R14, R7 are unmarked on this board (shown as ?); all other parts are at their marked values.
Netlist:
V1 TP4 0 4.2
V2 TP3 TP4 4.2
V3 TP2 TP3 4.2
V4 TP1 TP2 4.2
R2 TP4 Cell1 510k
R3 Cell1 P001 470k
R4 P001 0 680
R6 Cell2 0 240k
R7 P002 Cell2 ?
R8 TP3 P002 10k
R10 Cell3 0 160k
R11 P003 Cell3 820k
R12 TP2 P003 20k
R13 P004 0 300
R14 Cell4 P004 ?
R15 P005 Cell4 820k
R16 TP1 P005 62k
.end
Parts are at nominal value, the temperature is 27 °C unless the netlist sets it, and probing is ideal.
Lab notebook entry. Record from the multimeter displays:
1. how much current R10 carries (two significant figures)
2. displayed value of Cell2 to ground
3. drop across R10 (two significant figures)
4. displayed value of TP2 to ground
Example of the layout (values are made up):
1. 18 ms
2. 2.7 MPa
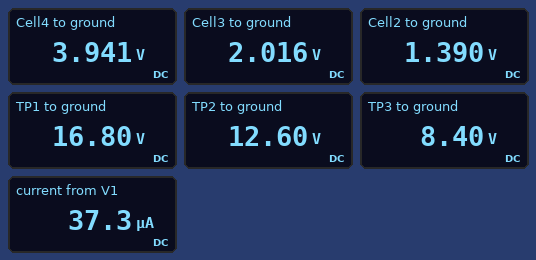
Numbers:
1. 13 µA
2. 1.390 V
3. 2.0 V
4. 12.60 V
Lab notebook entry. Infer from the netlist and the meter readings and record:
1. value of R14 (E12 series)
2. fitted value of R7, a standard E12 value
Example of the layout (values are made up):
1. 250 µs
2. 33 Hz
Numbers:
1. 270 kΩ
2. 1.2 MΩ
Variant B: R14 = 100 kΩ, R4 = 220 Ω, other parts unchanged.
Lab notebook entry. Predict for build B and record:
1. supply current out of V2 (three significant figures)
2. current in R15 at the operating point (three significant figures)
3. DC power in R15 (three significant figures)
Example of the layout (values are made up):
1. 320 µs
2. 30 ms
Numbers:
1. 35.5 µA
2. 17.1 µA
3. 240 µW
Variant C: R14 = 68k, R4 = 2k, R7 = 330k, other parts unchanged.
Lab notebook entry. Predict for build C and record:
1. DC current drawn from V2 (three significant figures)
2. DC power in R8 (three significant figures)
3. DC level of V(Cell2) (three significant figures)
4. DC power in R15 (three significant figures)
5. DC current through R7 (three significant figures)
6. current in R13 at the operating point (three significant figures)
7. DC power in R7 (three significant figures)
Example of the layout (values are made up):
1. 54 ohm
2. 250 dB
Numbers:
1. 44.8 µA
2. 2.10 µW
3. 3.48 V
4. 256 µW
5. 14.5 µA
6. 17.7 µA
7. 69.2 µW
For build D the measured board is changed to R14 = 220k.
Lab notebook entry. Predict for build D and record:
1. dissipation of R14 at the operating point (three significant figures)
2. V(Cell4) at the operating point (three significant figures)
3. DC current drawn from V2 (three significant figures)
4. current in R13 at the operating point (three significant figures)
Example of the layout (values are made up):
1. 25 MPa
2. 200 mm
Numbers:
1. 51.1 µW
2. 3.36 V
3. 33.6 µA
4. 15.2 µA
